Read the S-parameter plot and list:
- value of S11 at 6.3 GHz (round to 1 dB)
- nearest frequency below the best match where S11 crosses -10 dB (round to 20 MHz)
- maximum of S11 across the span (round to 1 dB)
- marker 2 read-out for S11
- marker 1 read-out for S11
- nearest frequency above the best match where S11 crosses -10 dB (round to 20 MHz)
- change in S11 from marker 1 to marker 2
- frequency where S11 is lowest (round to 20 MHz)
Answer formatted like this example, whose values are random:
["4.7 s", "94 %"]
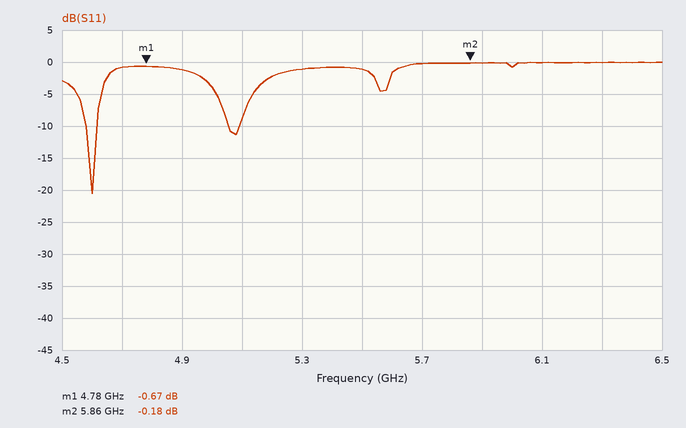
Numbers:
["0 dB", "4.58 GHz", "0 dB", "-0.18 dB", "-0.67 dB", "4.62 GHz", "0.49 dB", "4.60 GHz"]
